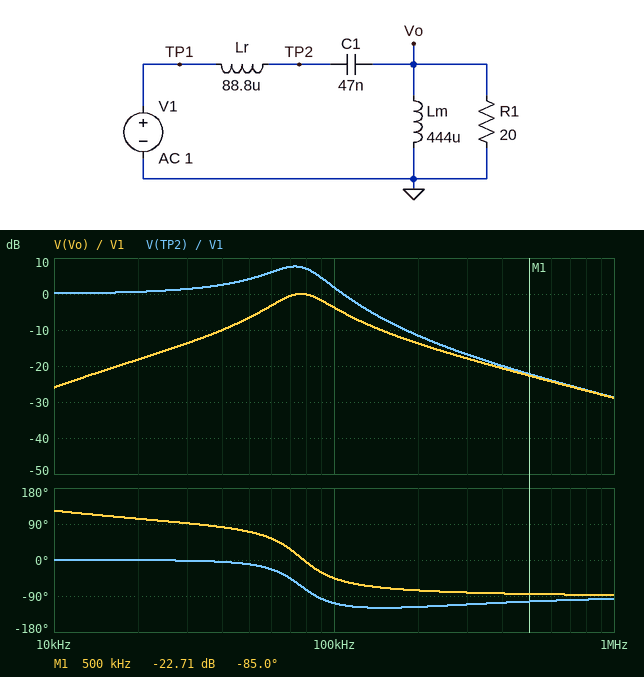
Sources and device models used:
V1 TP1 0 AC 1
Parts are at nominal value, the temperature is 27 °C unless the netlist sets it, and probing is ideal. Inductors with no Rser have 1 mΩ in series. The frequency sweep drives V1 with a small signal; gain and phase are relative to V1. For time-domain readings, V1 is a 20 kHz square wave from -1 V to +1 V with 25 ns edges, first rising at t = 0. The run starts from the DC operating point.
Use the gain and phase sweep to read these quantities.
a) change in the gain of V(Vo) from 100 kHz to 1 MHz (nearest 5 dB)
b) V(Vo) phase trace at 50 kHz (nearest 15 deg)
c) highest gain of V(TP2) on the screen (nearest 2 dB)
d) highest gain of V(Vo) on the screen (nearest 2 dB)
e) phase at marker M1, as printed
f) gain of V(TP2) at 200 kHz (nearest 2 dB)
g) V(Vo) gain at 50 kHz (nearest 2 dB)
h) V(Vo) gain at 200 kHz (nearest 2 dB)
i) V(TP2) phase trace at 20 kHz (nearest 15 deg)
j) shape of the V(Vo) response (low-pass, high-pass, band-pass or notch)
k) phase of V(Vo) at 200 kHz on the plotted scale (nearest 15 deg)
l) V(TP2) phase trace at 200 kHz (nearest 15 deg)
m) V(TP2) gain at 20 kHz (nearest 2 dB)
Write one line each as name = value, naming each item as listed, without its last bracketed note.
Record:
change in the gain of V(Vo) from 100 kHz to 1 MHz = -25 dB
V(Vo) phase trace at 50 kHz = 75 deg
highest gain of V(TP2) on the screen = 8 dB
highest gain of V(Vo) on the screen = 0 dB
phase at marker M1, as printed = -85.0 deg
gain of V(TP2) at 200 kHz = -12 dB
V(Vo) gain at 50 kHz = -6 dB
V(Vo) gain at 200 kHz = -14 dB
V(TP2) phase trace at 20 kHz = 0 deg
shape of the V(Vo) response = band-pass
phase of V(Vo) at 200 kHz on the plotted scale = -75 deg
V(TP2) phase trace at 200 kHz = -120 deg
V(TP2) gain at 20 kHz = 0 dB
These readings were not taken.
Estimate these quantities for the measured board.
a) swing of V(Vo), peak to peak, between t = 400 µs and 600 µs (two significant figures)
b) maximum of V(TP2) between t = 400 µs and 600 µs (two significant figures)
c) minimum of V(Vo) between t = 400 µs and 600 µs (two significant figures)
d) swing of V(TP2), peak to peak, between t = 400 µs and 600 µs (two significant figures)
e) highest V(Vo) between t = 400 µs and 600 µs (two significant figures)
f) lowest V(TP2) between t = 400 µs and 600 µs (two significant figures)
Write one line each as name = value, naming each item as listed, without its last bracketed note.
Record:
swing of V(Vo), peak to peak, between t = 400 µs and 600 µs = 1.3 V
maximum of V(TP2) between t = 400 µs and 600 µs = 2.0 V
minimum of V(Vo) between t = 400 µs and 600 µs = -630 mV
swing of V(TP2), peak to peak, between t = 400 µs and 600 µs = 4.1 V
highest V(Vo) between t = 400 µs and 600 µs = 630 mV
lowest V(TP2) between t = 400 µs and 600 µs = -2.0 V
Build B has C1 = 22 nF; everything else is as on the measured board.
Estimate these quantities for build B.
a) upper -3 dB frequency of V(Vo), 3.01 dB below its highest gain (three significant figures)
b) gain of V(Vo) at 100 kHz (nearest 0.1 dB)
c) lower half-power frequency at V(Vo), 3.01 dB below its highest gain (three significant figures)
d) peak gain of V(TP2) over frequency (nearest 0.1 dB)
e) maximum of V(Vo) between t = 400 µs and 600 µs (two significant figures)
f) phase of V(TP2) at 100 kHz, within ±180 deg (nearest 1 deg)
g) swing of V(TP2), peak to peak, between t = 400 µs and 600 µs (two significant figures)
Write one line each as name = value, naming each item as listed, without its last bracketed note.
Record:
upper -3 dB frequency of V(Vo), 3.01 dB below its highest gain = 132 kHz
gain of V(Vo) at 100 kHz = -2.0 dB
lower half-power frequency at V(Vo), 3.01 dB below its highest gain = 96.3 kHz
peak gain of V(TP2) over frequency = 10.5 dB
maximum of V(Vo) between t = 400 µs and 600 µs = 490 mV
phase of V(TP2) at 100 kHz, within ±180 deg = -37 deg
swing of V(TP2), peak to peak, between t = 400 µs and 600 µs = 4.5 V
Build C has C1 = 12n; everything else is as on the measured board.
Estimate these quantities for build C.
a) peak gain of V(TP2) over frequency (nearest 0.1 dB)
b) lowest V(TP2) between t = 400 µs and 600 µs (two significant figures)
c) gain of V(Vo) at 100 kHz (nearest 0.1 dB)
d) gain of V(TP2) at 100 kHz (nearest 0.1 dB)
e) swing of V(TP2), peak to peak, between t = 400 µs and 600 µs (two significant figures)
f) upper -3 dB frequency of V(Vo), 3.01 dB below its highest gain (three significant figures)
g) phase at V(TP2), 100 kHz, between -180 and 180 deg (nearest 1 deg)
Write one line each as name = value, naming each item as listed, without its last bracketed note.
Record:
peak gain of V(TP2) over frequency = 12.9 dB
lowest V(TP2) between t = 400 µs and 600 µs = -2.4 V
gain of V(Vo) at 100 kHz = -11.8 dB
gain of V(TP2) at 100 kHz = 4.6 dB
swing of V(TP2), peak to peak, between t = 400 µs and 600 µs = 4.8 V
upper -3 dB frequency of V(Vo), 3.01 dB below its highest gain = 172 kHz
phase at V(TP2), 100 kHz, between -180 and 180 deg = -6 deg
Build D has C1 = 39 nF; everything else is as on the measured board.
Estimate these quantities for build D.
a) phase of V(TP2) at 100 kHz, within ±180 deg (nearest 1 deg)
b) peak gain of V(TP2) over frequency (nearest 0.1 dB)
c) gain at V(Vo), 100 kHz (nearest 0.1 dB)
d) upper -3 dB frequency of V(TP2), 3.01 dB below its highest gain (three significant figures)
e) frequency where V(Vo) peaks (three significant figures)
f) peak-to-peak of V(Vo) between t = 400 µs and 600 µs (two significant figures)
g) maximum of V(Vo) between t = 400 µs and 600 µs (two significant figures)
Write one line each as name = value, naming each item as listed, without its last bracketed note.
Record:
phase of V(TP2) at 100 kHz, within ±180 deg = -103 deg
peak gain of V(TP2) over frequency = 8.3 dB
gain at V(Vo), 100 kHz = -2.2 dB
upper -3 dB frequency of V(TP2), 3.01 dB below its highest gain = 97.6 kHz
frequency where V(Vo) peaks = 84.0 kHz
peak-to-peak of V(Vo) between t = 400 µs and 600 µs = 1.1 V
maximum of V(Vo) between t = 400 µs and 600 µs = 570 mV
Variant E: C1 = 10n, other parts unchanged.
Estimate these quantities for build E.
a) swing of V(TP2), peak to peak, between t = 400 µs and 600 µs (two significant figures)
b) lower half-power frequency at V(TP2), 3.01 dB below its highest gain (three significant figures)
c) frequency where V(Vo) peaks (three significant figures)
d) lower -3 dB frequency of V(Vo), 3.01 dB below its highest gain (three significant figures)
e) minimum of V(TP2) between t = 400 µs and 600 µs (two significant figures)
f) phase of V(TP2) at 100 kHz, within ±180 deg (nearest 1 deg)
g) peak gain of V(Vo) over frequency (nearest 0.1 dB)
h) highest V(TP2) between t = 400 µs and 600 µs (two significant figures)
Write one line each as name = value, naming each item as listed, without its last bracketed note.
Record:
swing of V(TP2), peak to peak, between t = 400 µs and 600 µs = 4.8 V
lower half-power frequency at V(TP2), 3.01 dB below its highest gain = 147 kHz
frequency where V(Vo) peaks = 168 kHz
lower -3 dB frequency of V(Vo), 3.01 dB below its highest gain = 151 kHz
minimum of V(TP2) between t = 400 µs and 600 µs = -2.4 V
phase of V(TP2) at 100 kHz, within ±180 deg = -4 deg
peak gain of V(Vo) over frequency = 0 dB
highest V(TP2) between t = 400 µs and 600 µs = 2.4 V
